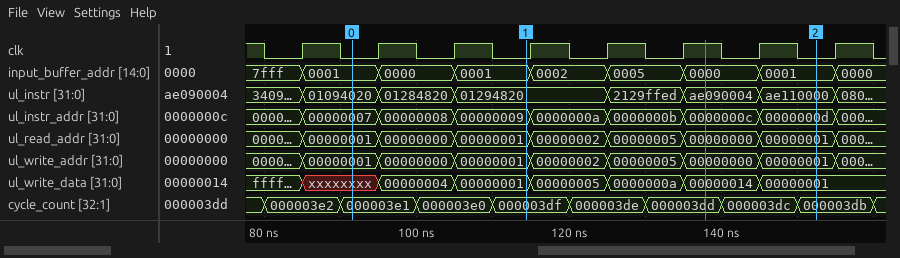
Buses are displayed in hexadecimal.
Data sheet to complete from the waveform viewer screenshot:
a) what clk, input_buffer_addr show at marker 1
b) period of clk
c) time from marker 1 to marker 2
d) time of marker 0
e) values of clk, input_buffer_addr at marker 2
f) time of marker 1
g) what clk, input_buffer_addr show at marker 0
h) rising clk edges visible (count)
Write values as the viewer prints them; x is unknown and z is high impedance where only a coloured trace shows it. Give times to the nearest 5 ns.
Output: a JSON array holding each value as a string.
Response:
["clk=0, input_buffer_addr=0001", "10 ns", "40 ns", "90 ns", "clk=0, input_buffer_addr=0001", "115 ns", "clk=0, input_buffer_addr=0001", "8"]
